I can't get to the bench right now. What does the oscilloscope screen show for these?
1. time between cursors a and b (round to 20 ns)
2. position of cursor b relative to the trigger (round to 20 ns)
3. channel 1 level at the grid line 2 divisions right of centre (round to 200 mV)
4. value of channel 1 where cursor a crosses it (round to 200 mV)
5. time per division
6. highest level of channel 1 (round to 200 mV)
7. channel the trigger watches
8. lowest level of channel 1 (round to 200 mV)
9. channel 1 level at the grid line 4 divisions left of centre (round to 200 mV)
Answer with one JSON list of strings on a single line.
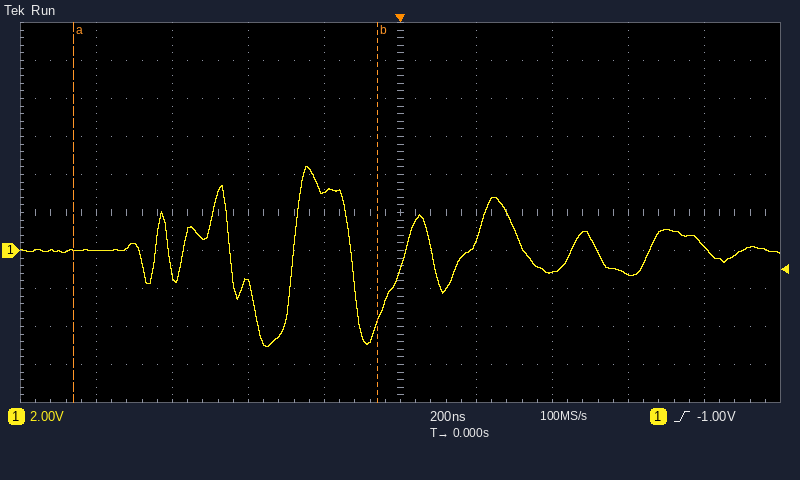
["800 ns", "-60 ns", "-1.2 V", "0.0 V", "200 ns", "4.4 V", "channel 1", "-5.0 V", "0.0 V"]
